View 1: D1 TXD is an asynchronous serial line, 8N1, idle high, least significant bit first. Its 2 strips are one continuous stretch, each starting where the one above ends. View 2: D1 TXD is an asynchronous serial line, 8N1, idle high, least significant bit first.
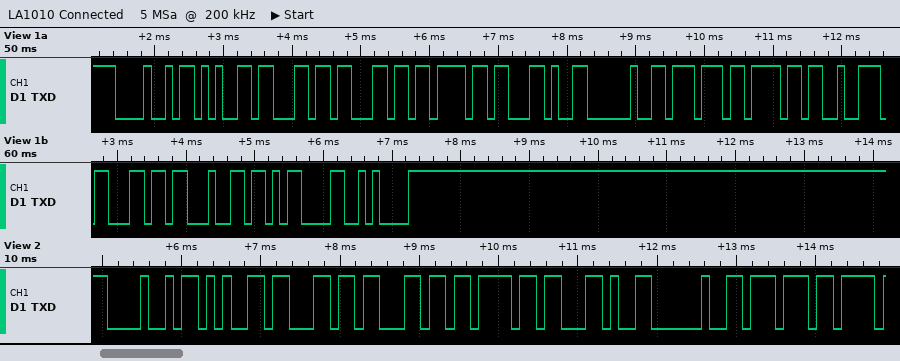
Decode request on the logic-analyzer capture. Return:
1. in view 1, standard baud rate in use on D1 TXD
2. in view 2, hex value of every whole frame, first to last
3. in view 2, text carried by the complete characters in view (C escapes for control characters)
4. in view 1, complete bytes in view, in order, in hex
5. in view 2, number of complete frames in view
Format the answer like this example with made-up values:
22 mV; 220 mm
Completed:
9600 baud; 48 65 6C 6C 6F 2C 20 77; "Hello, w"; 48 65 6C 6C 6F 2C 20 77 6F 72 6C 64 0D 0A; 8
